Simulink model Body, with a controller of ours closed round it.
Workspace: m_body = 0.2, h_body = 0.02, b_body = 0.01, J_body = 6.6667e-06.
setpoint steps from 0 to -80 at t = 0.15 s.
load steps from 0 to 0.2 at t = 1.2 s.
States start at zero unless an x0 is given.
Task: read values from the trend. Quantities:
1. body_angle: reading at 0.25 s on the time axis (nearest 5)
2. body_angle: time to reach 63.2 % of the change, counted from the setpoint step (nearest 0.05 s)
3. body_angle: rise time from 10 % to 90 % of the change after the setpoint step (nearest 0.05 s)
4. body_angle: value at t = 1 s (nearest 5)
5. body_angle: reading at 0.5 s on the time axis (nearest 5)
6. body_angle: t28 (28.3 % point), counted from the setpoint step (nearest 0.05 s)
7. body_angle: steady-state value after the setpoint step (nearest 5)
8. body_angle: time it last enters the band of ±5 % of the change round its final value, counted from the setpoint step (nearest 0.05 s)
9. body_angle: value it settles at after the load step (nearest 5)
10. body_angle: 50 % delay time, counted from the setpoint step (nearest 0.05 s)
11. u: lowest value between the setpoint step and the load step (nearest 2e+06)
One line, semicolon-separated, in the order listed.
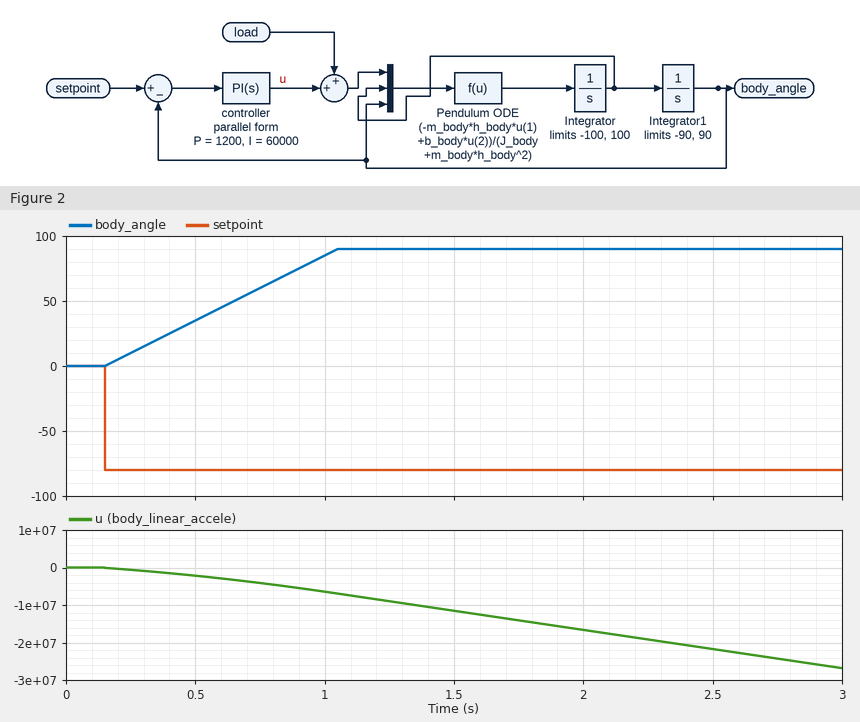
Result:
10; 0.55 s; 0.70 s; 85; 35; 0.25 s; 90; 0.85 s; 90; 0.45 s; -8000000
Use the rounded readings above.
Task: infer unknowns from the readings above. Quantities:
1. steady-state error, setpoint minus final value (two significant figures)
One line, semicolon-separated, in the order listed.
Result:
-170
